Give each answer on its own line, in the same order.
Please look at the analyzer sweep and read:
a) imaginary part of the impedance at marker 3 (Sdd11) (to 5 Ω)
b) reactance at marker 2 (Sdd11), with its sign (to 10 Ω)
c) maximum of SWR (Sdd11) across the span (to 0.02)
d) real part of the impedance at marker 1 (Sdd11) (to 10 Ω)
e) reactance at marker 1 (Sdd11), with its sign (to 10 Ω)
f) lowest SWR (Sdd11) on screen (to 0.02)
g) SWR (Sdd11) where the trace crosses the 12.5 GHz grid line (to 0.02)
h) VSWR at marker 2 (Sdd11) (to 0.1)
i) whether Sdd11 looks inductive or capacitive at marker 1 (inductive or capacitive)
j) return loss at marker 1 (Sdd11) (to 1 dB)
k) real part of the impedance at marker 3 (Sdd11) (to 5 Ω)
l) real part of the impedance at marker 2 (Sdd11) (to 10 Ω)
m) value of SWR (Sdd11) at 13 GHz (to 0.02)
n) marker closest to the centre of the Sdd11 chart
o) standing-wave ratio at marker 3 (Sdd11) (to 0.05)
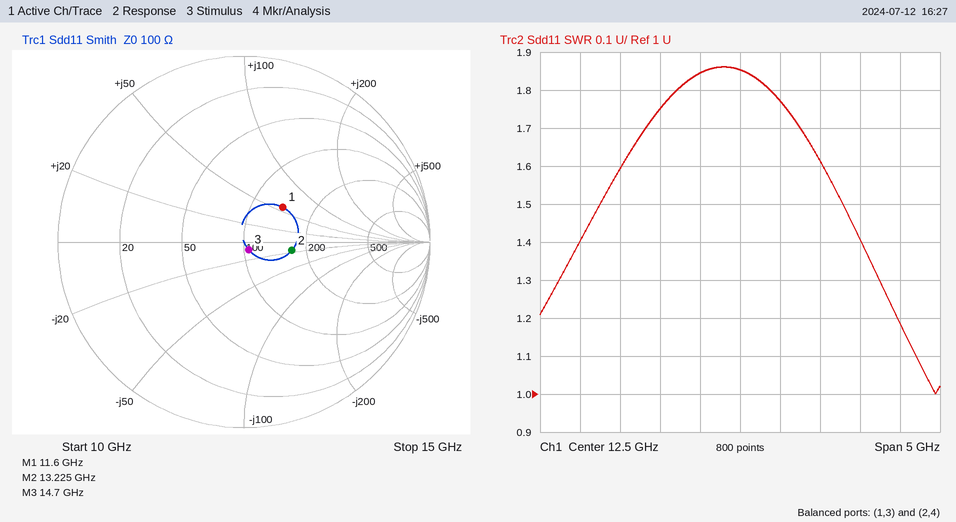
-10 Ω
-20 Ω
1.86
140 Ω
+60 Ω
1.00
1.86
1.7
inductive
11 dB
105 Ω
170 Ω
1.78
marker 3
1.10
